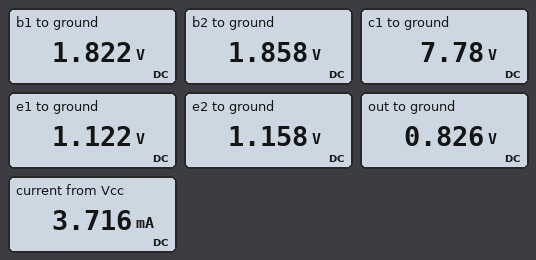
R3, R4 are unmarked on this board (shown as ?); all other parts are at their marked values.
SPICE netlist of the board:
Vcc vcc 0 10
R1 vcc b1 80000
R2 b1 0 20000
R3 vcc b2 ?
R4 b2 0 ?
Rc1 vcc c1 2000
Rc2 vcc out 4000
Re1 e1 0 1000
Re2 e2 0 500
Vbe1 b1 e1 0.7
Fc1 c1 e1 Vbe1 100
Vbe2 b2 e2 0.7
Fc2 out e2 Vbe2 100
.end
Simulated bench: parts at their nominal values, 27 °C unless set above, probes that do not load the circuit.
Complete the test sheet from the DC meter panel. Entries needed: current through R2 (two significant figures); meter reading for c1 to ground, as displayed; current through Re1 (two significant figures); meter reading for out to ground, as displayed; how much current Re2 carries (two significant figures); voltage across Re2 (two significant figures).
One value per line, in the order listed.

91 µA
7.78 V
1.1 mA
0.826 V
2.3 mA
1.2 V
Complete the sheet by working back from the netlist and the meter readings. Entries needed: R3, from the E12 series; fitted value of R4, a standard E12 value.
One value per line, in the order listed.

39 kΩ
10 kΩ
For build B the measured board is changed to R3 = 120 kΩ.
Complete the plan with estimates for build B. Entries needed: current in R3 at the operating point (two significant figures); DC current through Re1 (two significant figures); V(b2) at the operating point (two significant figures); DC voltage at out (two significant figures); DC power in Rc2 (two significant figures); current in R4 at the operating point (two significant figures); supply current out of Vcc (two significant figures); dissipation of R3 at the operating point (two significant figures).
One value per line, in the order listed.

77 µA
1.1 mA
760 mV
9.5 V
54 µW
76 µA
1.4 mA
710 µW
